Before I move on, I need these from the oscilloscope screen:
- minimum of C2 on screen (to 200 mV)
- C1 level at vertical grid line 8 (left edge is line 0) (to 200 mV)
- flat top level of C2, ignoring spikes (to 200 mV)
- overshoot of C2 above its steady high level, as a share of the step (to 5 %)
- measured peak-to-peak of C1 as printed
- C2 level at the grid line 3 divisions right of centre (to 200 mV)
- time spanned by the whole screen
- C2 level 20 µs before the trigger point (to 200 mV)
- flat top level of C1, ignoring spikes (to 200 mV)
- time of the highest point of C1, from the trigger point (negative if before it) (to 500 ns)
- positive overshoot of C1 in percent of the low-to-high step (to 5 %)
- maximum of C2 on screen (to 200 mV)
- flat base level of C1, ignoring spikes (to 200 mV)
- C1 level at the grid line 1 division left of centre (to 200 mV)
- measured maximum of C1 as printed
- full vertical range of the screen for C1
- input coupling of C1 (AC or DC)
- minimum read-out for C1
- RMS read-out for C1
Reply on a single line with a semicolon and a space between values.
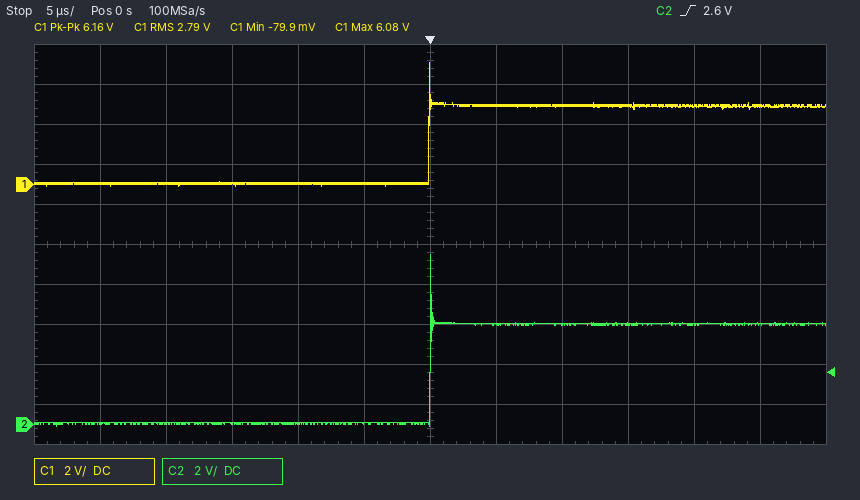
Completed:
0.0 V; 4.0 V; 5.0 V; 70 %; 6.16 V; 5.0 V; 60 µs; 0.0 V; 4.0 V; 0.0 µs; 55 %; 8.4 V; 0.0 V; 0.0 V; 6.08 V; 20 V; DC; -79.9 mV; 2.79 V
